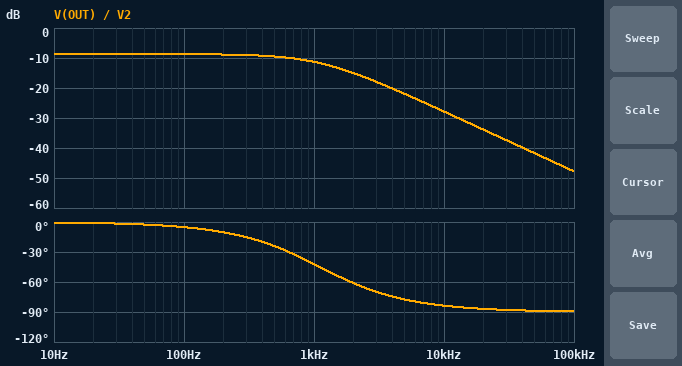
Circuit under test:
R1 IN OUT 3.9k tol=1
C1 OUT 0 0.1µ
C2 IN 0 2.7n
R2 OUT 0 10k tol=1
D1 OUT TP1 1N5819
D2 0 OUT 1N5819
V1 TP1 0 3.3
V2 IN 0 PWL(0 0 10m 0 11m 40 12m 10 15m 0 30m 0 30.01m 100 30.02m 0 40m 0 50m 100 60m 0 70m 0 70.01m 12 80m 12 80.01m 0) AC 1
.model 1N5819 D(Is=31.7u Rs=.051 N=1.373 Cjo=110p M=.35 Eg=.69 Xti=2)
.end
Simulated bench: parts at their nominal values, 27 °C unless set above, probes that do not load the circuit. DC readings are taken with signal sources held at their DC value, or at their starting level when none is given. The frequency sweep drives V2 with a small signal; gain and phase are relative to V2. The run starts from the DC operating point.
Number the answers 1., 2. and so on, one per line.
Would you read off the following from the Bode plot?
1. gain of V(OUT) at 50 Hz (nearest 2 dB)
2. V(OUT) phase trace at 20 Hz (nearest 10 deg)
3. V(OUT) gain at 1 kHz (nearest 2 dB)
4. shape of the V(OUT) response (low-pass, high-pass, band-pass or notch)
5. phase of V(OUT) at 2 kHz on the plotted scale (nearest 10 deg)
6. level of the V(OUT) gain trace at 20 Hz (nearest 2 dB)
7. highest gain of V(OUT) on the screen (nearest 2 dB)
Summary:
1. -8 dB
2. 0 deg
3. -12 dB
4. low-pass
5. -60 deg
6. -8 dB
7. -8 dB
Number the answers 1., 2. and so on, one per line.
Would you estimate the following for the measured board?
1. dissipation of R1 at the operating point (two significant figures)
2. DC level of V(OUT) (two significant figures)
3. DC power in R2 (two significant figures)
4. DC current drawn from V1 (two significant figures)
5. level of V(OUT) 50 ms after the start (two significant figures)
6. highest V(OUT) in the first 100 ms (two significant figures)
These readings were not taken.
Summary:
1. 300 nW
2. 34 mV
3. 120 nW
4. 32 µA
5. 3.5 V
6. 3.5 V
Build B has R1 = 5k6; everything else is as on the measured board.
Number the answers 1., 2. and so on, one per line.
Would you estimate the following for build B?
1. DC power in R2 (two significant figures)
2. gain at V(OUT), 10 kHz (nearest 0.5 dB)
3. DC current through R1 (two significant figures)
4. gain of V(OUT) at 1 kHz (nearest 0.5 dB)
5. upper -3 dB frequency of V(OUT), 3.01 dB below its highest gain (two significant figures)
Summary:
1. 150 nW
2. -31.0 dB
3. 6.9 µA
4. -13.5 dB
5. 920 Hz
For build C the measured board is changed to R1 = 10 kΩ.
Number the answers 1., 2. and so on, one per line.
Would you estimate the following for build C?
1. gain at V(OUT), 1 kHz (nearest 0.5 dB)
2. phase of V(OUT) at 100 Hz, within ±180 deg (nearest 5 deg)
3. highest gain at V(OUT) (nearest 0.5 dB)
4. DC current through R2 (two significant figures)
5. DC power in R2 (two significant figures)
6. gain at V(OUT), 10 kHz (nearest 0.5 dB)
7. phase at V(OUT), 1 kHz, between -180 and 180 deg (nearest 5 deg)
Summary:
1. -18.0 dB
2. -10 deg
3. -13.0 dB
4. 4.5 µA
5. 200 nW
6. -36.0 dB
7. -55 deg
